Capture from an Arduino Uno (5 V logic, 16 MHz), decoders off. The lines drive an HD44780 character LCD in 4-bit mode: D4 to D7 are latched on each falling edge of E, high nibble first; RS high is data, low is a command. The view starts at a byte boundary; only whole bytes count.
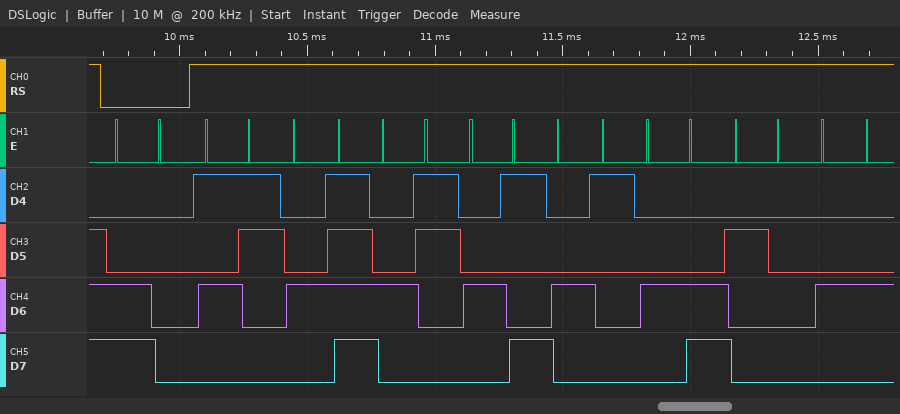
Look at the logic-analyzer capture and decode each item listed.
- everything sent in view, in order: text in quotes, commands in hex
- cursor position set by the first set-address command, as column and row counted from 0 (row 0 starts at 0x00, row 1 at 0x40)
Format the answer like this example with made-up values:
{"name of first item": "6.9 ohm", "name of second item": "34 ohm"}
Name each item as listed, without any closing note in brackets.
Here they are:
{"everything sent in view, in order: text in quotes, commands in hex": "0xC0 \"SOCIAL D\"", "cursor position set by the first set-address command, as column and row counted from 0": "column 0, row 1"}
